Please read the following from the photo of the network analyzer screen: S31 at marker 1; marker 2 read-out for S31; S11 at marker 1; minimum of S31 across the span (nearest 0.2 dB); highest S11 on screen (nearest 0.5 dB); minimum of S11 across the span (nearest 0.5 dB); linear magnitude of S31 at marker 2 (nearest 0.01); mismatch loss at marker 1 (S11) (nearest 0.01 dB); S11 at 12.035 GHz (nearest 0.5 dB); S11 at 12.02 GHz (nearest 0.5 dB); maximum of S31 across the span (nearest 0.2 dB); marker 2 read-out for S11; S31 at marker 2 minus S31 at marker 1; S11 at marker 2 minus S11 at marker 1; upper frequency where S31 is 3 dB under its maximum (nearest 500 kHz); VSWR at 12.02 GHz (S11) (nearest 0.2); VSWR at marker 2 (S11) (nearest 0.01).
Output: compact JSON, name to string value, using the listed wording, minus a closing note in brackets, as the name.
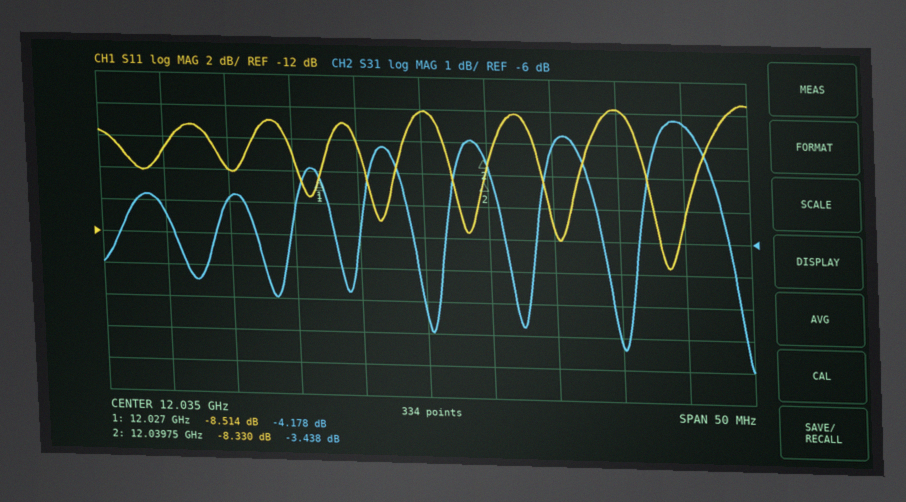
{"S31 at marker 1": "-4.178 dB", "marker 2 read-out for S31": "-3.438 dB", "S11 at marker 1": "-8.514 dB", "minimum of S31 across the span": "-10.0 dB", "highest S11 on screen": "-3.5 dB", "minimum of S11 across the span": "-13.5 dB", "linear magnitude of S31 at marker 2": "0.67", "mismatch loss at marker 1 (S11)": "0.66 dB", "S11 at 12.035 GHz": "-4.0 dB", "S11 at 12.02 GHz": "-8.0 dB", "maximum of S31 across the span": "-2.2 dB", "marker 2 read-out for S11": "-8.330 dB", "S31 at marker 2 minus S31 at marker 1": "0.740 dB", "S11 at marker 2 minus S11 at marker 1": "0.184 dB", "upper frequency where S31 is 3 dB under its maximum": "12.0580 GHz", "VSWR at 12.02 GHz (S11)": "2.4", "VSWR at marker 2 (S11)": "2.24"}
